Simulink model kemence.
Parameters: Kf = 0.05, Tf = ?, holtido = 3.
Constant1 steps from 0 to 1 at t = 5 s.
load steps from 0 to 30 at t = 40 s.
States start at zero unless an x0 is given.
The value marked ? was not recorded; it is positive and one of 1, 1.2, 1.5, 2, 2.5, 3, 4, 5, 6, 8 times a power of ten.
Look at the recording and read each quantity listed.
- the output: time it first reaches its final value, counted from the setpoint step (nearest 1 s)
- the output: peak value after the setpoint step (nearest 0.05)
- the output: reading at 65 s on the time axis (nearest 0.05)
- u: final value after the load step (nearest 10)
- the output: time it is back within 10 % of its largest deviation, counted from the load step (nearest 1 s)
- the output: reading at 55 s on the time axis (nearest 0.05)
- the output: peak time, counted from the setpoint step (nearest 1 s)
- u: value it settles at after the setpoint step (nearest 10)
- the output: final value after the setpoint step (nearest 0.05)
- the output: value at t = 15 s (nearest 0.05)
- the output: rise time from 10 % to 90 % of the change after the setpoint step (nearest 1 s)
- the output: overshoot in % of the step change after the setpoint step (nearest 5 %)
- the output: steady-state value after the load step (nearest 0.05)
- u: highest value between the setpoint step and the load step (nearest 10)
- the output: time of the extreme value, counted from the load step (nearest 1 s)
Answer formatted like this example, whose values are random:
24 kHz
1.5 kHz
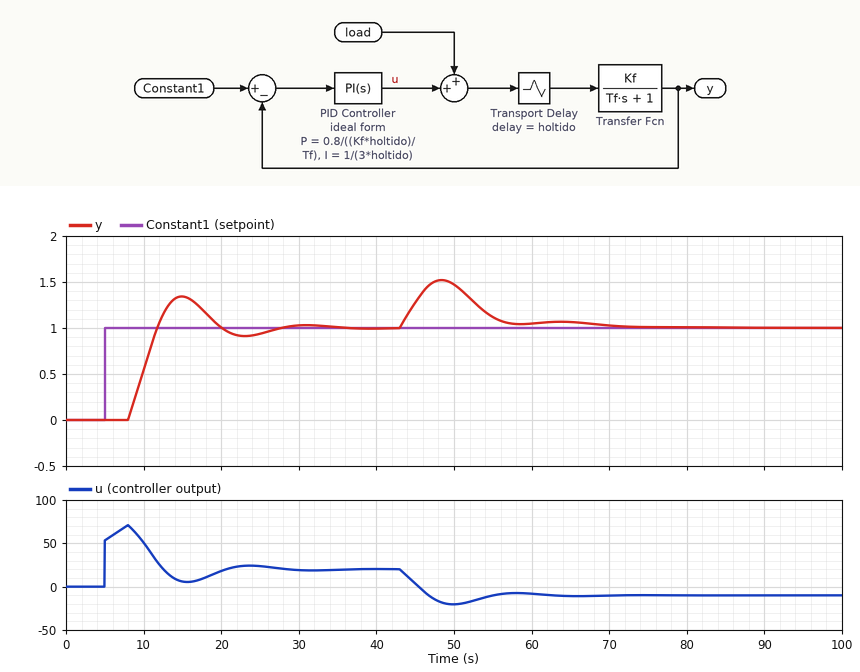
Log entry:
7 s
1.35
1.05
-10
27 s
1.10
10 s
20
1.00
1.35
3 s
35 %
1.00
70
8 s
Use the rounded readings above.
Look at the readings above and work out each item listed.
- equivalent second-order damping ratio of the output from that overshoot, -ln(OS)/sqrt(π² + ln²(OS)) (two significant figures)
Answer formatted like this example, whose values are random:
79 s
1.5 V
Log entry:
0.32
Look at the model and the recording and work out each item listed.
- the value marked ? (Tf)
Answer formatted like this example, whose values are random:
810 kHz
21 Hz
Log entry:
10
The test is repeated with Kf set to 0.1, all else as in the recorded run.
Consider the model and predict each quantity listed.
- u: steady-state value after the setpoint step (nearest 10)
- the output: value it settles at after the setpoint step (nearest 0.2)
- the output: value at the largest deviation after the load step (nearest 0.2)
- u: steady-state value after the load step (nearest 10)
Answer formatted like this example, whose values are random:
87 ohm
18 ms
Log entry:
10
1.0
2.0
-20
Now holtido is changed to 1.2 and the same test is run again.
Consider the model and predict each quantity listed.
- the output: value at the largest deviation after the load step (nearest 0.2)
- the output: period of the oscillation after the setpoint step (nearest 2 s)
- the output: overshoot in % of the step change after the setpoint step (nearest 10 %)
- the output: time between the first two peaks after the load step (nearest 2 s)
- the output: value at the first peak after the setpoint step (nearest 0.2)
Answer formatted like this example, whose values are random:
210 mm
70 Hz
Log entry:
1.2
8 s
60 %
8 s
1.6
